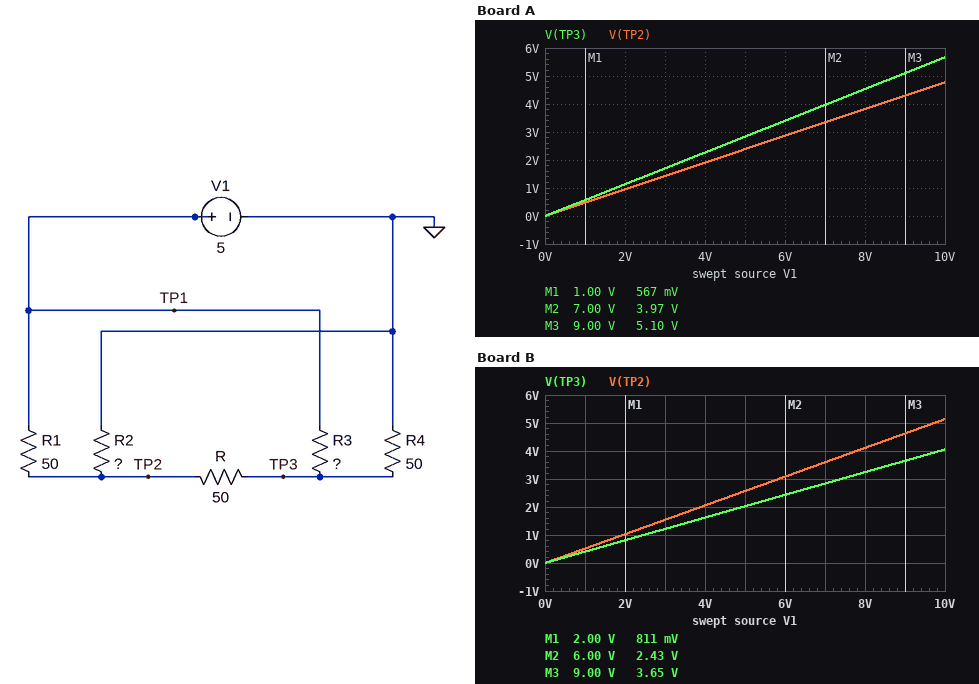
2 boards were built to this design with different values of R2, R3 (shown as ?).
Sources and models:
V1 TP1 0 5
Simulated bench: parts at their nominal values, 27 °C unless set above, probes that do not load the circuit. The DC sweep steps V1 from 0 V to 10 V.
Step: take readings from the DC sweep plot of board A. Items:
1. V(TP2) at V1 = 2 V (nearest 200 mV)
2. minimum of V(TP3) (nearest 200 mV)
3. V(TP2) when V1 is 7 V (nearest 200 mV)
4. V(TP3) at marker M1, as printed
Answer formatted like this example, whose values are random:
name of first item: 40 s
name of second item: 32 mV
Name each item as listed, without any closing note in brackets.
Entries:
V(TP2) at V1 = 2 V: 1.0 V
minimum of V(TP3): 0 V
V(TP2) when V1 is 7 V: 3.4 V
V(TP3) at marker M1, as printed: 567 mV
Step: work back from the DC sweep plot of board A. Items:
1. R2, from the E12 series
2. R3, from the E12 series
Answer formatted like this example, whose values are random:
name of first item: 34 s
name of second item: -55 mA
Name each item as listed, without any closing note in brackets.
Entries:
R2, from the E12 series: 39 Ω
R3, from the E12 series: 33 Ω
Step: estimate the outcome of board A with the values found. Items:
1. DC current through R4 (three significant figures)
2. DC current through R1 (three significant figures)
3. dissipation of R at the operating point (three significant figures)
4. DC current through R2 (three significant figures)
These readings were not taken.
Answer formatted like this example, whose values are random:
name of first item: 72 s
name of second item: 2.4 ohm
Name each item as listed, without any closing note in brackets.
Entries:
DC current through R4: 56.7 mA
DC current through R1: 52.3 mA
dissipation of R at the operating point: 4.00 mW
DC current through R2: 61.2 mA
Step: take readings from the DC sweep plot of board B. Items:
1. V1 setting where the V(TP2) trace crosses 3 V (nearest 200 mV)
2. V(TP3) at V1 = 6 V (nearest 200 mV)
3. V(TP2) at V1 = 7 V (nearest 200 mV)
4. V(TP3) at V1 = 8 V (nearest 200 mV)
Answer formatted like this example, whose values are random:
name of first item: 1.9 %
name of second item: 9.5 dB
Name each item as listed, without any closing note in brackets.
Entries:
V1 setting where the V(TP2) trace crosses 3 V: 5.8 V
V(TP3) at V1 = 6 V: 2.4 V
V(TP2) at V1 = 7 V: 3.6 V
V(TP3) at V1 = 8 V: 3.2 V
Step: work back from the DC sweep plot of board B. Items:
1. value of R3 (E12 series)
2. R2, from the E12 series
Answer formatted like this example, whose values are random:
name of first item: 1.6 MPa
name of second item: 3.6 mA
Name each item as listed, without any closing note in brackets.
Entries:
value of R3: 100 Ω
R2, from the E12 series: 68 Ω
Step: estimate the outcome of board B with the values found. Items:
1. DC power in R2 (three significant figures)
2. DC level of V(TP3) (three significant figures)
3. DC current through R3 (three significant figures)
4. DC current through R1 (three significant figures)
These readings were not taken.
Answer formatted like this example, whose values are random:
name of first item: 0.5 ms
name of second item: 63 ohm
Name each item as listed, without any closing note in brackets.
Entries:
DC power in R2: 97.1 mW
DC level of V(TP3): 2.03 V
DC current through R3: 29.7 mA
DC current through R1: 48.6 mA
